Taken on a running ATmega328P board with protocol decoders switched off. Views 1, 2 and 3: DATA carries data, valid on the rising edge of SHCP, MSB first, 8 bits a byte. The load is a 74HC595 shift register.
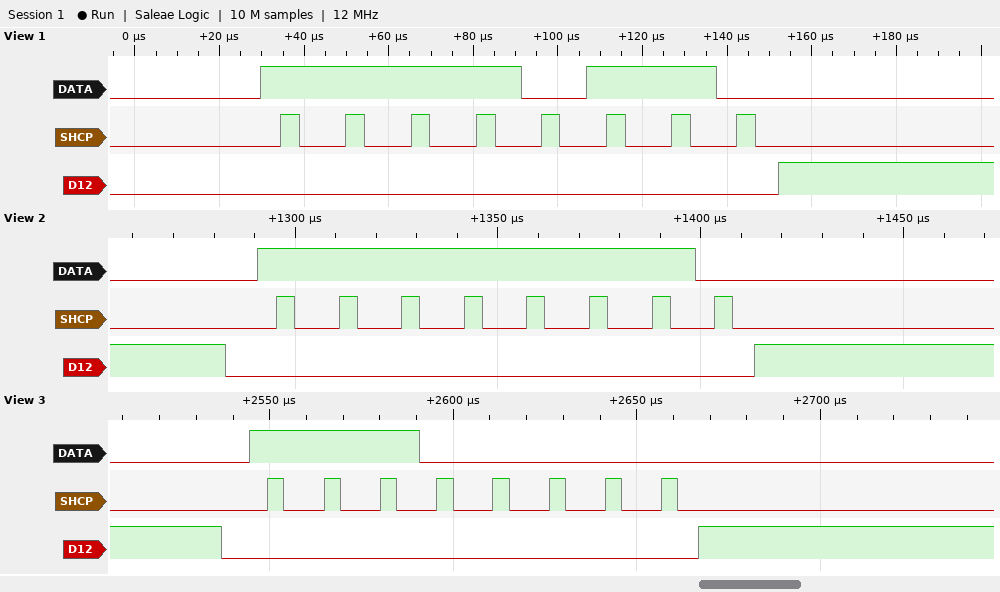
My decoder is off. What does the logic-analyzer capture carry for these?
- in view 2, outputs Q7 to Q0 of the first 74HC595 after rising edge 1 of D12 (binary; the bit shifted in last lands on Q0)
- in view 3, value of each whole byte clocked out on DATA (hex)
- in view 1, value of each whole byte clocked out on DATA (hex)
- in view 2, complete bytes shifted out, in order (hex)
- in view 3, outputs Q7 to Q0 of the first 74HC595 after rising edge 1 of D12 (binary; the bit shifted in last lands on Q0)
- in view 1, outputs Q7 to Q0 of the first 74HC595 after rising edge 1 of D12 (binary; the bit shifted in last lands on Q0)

11111110
0xE0
F6
0xFE
11100000
11110110
